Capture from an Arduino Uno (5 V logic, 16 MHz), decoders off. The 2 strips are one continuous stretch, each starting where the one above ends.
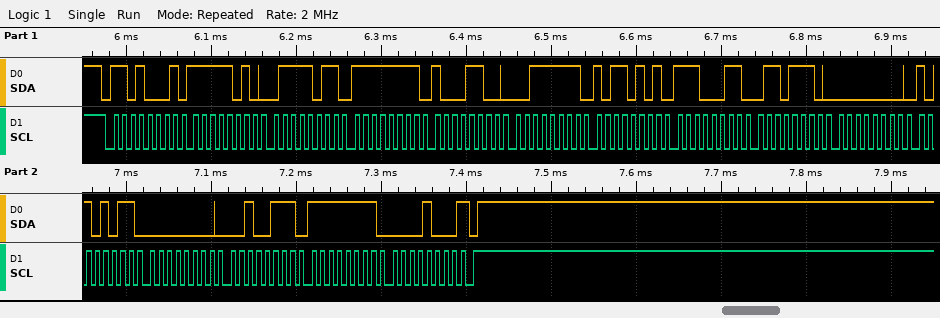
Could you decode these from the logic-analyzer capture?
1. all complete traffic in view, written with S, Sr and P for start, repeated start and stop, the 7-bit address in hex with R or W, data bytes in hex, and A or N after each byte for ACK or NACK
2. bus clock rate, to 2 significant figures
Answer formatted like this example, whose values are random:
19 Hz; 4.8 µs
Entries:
S 68R A FA A 7B A FF A 8C A 3F A B5 A E3 A 6E A 00 A AB A 00 A 27 A FF A 08 N P; 100 kHz
